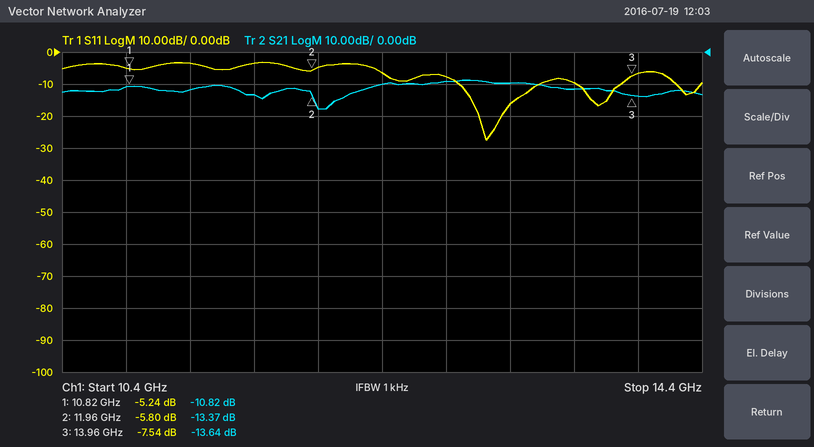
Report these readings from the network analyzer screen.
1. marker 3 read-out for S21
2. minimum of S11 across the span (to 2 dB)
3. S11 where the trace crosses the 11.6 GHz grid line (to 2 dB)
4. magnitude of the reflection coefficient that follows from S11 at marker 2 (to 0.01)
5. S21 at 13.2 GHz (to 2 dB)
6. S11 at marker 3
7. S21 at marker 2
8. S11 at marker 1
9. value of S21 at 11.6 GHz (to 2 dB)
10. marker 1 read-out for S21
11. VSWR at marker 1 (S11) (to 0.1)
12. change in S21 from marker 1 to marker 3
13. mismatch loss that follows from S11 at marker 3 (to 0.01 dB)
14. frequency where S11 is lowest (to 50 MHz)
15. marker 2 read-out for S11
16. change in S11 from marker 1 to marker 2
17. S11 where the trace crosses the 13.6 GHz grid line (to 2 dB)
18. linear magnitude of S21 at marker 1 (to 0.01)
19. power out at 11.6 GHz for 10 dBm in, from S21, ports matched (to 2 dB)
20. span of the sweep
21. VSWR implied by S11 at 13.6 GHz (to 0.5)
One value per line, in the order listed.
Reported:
-13.64 dB
-28 dB
-4 dB
0.51
-10 dB
-7.54 dB
-13.37 dB
-5.24 dB
-14 dB
-10.82 dB
3.4
-2.82 dB
0.84 dB
13.05 GHz
-5.80 dB
-0.56 dB
-10 dB
0.29
-4 dBm
4 GHz
2.0
